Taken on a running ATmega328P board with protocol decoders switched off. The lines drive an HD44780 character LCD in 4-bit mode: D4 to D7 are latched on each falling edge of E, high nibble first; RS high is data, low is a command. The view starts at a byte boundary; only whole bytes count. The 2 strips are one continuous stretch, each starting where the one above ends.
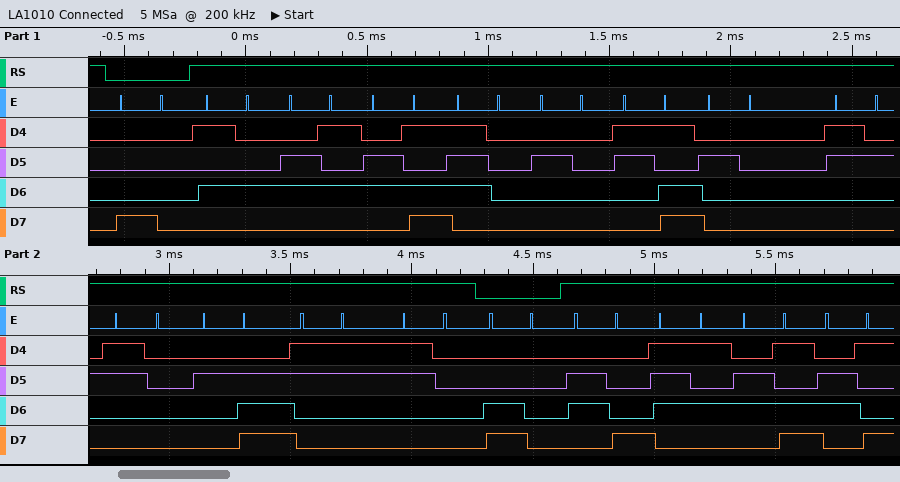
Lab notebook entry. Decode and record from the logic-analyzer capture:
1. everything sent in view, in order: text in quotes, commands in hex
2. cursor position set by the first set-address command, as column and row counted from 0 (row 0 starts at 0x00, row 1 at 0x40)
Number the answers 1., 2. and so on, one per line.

1. 0x80 "Temp = 20.30" 0xC0 "humi"
2. column 0, row 0
